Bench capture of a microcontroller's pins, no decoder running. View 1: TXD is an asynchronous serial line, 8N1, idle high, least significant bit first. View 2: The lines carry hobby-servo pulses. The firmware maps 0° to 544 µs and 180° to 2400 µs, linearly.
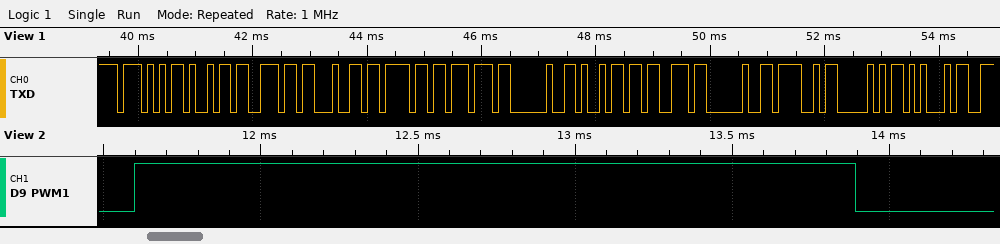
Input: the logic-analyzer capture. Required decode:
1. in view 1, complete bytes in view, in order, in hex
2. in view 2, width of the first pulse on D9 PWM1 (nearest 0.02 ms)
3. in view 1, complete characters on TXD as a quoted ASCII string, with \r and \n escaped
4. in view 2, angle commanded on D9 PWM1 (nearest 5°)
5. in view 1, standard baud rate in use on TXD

0x57 0x69 0x6E 0x64 0x6F 0x77 0x20 0x69 0x73 0x20 0x4F 0x50 0x45
2.30 ms
"Window is OPE"
170°
9600 baud
